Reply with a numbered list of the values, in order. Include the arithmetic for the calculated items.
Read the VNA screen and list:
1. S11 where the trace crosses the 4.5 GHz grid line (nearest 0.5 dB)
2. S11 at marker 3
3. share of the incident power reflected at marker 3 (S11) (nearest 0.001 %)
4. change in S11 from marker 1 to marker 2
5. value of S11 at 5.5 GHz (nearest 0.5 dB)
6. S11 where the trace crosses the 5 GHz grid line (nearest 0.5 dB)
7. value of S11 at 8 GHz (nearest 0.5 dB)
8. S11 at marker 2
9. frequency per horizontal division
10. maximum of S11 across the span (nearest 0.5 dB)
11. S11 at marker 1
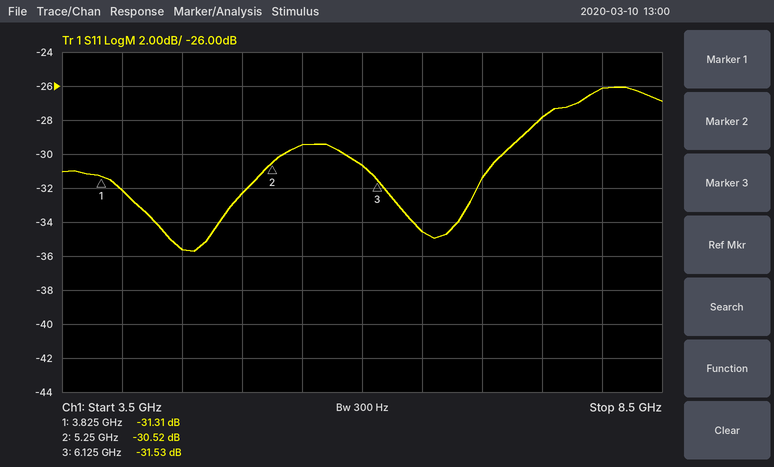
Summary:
1. -35.5 dB
2. -31.53 dB
3. 10^(-31.53/10) ≈ 0.070 %
4. -30.52 − (-31.31) = 0.79 dB
5. -29.5 dB
6. -32.5 dB
7. -26.0 dB
8. -30.52 dB
9. 500 MHz
10. -26.0 dB
11. -31.31 dB
